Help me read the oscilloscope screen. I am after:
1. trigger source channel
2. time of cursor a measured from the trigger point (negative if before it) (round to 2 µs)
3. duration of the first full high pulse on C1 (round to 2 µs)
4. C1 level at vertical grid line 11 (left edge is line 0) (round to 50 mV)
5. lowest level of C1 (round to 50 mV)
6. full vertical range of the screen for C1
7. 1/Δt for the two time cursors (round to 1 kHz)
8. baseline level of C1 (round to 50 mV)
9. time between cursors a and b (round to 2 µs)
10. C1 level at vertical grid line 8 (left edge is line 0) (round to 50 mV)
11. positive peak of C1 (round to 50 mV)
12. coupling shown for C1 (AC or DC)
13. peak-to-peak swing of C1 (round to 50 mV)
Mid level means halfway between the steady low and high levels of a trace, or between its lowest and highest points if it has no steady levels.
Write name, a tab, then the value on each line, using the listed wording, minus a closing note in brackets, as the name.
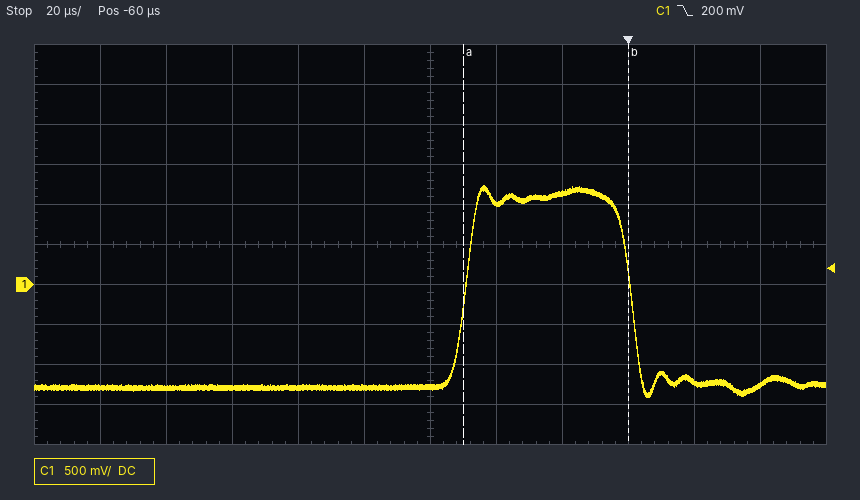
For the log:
trigger source channel	C1
time of cursor a measured from the trigger point (negative if before it)	-50 µs
duration of the first full high pulse on C1	50 µs
C1 level at vertical grid line 11 (left edge is line 0)	-1.25 V
lowest level of C1	-1.40 V
full vertical range of the screen for C1	5 V
1/Δt for the two time cursors	20 kHz
baseline level of C1	-1.30 V
time between cursors a and b	50 µs
C1 level at vertical grid line 8 (left edge is line 0)	1.15 V
positive peak of C1	1.25 V
coupling shown for C1	DC
peak-to-peak swing of C1	2.65 V
